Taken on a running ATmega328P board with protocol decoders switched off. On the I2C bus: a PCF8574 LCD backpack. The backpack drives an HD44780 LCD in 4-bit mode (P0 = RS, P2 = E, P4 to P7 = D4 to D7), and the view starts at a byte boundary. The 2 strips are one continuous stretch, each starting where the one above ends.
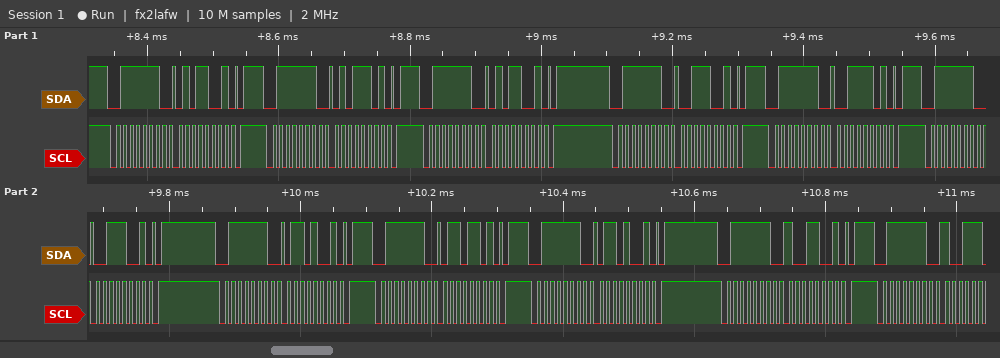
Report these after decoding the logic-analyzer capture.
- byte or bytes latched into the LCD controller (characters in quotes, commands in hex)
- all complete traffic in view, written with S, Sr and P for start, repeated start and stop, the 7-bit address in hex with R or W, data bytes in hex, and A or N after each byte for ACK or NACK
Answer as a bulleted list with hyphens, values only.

- 'S'
- S 3FW A 59 A P S 3FW A 5D A P S 3FW A 59 A P S 3FW A 39 A P S 3FW A 3D A P S 3FW A 39 A P S 3FW A 69 A P S 3FW A 6D A P S 3FW A 69 A P S 3FW A 99 A P S 3FW A
